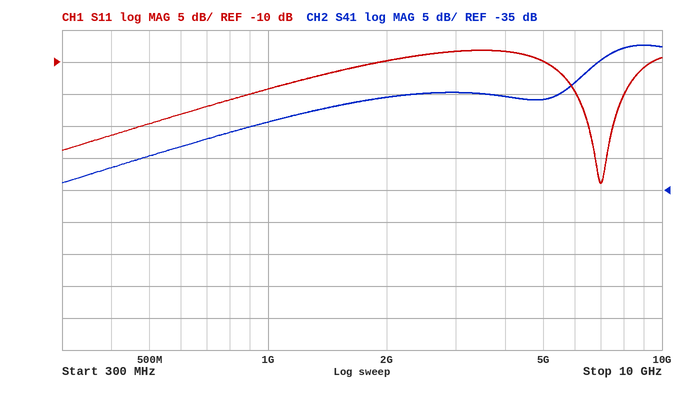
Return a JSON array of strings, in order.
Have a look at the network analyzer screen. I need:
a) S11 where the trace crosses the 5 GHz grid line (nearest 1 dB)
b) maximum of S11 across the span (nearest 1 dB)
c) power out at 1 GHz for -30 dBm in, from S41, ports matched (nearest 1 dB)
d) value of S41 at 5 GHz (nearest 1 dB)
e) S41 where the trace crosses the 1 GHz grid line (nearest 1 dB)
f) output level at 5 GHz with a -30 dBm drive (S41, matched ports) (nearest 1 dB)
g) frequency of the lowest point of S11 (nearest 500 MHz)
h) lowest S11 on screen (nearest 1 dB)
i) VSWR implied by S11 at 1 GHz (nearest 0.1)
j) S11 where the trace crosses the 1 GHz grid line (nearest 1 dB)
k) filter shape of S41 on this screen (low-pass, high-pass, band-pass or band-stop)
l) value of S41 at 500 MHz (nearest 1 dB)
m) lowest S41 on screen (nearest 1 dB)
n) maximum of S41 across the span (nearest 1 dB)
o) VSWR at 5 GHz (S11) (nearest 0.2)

["-10 dB", "-8 dB", "-54 dBm", "-21 dB", "-24 dB", "-51 dBm", "7.0 GHz", "-29 dB", "1.5", "-14 dB", "high-pass", "-30 dB", "-34 dB", "-12 dB", "2.0"]
